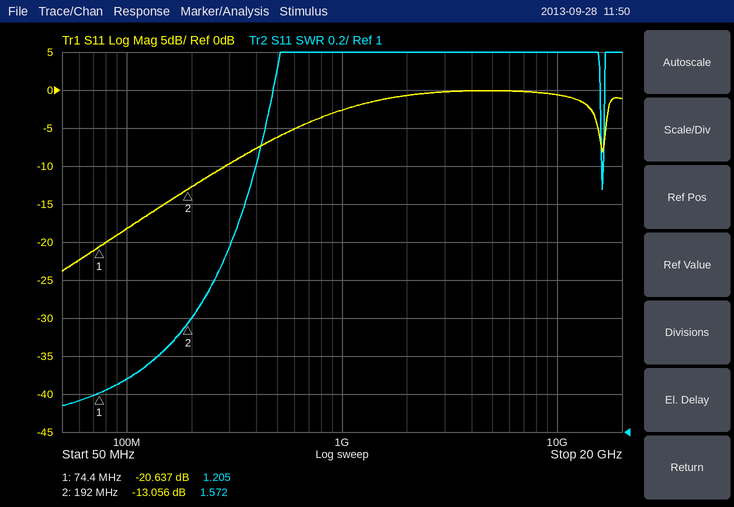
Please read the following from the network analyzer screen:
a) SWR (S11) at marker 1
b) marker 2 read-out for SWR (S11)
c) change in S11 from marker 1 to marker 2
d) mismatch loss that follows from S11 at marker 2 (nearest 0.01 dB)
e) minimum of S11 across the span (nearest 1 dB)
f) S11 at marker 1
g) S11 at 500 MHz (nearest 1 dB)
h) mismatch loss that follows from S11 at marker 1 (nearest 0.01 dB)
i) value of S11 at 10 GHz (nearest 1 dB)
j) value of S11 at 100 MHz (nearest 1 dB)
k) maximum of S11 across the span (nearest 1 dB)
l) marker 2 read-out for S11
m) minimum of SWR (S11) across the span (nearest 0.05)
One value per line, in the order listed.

1.205
1.572
7.581 dB
0.22 dB
-24 dB
-20.637 dB
-6 dB
0.04 dB
-1 dB
-18 dB
0 dB
-13.056 dB
1.15
